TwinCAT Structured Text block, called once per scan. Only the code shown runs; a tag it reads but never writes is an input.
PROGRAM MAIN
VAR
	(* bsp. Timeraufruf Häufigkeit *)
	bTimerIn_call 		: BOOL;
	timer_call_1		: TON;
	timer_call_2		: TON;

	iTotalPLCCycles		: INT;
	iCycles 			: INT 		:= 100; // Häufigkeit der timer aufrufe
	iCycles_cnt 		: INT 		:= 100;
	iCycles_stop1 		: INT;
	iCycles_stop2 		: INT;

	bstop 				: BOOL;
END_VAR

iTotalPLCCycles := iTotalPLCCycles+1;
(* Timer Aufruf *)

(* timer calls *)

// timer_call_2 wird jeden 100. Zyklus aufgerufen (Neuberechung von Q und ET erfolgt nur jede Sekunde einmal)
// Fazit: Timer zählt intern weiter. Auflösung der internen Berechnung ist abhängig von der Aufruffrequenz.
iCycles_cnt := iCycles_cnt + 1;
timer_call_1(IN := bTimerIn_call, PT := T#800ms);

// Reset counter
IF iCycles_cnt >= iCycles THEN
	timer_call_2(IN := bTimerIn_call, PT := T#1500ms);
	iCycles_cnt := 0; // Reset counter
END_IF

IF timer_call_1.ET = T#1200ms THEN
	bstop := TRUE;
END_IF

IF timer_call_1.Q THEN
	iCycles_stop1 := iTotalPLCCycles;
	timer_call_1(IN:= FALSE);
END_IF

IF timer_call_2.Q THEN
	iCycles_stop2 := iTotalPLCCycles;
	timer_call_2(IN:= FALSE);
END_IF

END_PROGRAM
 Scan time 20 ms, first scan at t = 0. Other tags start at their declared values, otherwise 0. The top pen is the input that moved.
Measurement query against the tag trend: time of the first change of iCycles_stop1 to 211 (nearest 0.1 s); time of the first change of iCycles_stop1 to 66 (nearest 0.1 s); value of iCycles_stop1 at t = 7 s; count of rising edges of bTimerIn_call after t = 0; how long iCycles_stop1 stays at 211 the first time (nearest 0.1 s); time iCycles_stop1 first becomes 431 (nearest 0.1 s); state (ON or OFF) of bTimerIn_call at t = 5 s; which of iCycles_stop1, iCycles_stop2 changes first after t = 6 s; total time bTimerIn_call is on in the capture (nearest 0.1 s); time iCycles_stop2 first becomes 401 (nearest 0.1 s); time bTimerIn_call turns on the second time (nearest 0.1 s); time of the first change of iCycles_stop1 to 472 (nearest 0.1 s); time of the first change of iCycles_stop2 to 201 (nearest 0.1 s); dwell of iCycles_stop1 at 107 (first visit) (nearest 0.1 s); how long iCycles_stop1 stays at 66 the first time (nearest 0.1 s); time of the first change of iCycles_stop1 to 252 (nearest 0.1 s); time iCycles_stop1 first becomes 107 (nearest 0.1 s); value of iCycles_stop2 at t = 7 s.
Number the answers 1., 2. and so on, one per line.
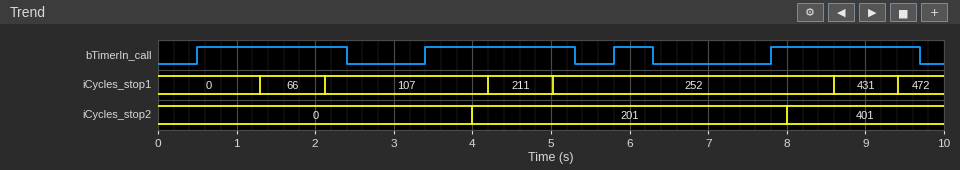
1. 4.2 s
2. 1.3 s
3. 252
4. 4
5. 0.8 s
6. 8.6 s
7. ON
8. iCycles_stop2
9. 6.2 s
10. 8.0 s
11. 3.4 s
12. 9.4 s
13. 4.0 s
14. 2.1 s
15. 0.8 s
16. 5.0 s
17. 2.1 s
18. 201
